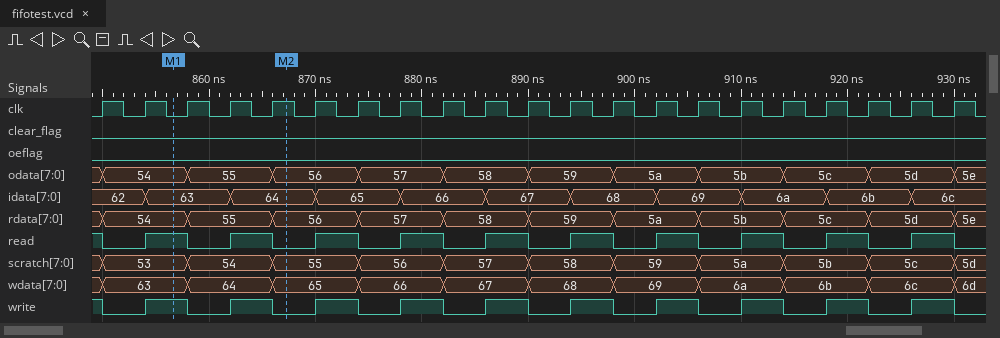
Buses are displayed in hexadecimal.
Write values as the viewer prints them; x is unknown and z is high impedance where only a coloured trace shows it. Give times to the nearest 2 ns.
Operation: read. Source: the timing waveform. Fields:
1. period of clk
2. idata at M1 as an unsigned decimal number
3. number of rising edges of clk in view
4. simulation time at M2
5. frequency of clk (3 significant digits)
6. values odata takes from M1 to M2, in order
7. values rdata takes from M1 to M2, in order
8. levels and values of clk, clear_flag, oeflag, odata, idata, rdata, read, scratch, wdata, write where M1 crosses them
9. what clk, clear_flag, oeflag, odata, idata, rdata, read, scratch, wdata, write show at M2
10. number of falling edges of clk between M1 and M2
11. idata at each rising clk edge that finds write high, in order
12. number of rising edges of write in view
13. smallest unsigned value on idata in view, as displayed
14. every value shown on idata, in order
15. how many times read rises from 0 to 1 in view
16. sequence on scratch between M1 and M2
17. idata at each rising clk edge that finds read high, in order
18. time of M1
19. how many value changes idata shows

4 ns
99
21
868 ns
250 MHz
54, 55, 56
54, 55, 56
clk=0, clear_flag=0, oeflag=0, odata=54, idata=63, rdata=54, read=1, scratch=53, wdata=63, write=1
clk=1, clear_flag=0, oeflag=0, odata=56, idata=64, rdata=56, read=0, scratch=55, wdata=65, write=0
2
62, 63, 64, 65, 66, 67, 68, 69, 6a, 6b, 6c
10
62
62, 63, 64, 65, 66, 67, 68, 69, 6a, 6b, 6c
10
53, 54, 55
62, 63, 64, 65, 66, 67, 68, 69, 6a, 6b, 6c
856 ns
10
